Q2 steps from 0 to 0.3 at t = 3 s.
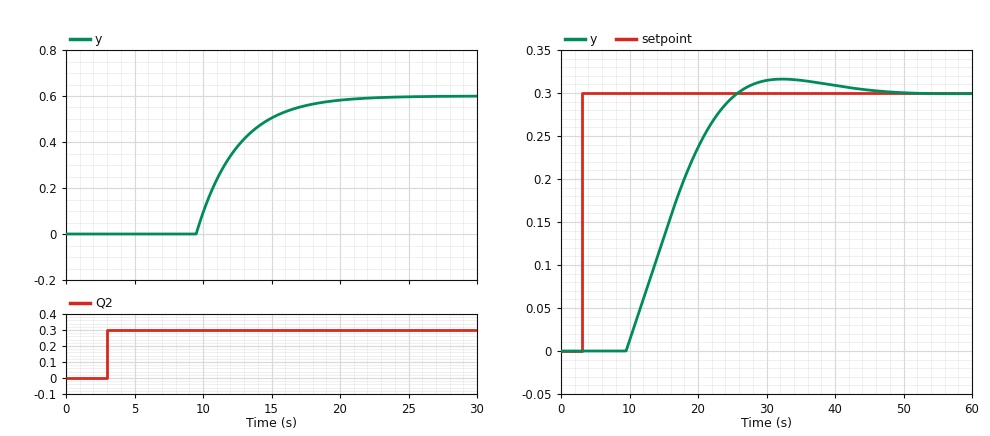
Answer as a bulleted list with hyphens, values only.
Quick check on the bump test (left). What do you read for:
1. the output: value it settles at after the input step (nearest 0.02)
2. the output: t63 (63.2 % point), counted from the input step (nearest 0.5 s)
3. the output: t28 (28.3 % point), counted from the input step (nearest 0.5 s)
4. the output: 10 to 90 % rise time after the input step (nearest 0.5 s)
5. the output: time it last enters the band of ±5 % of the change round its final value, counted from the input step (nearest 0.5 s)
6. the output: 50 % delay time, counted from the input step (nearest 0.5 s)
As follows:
- 0.60
- 9.5 s
- 7.5 s
- 6.5 s
- 15.5 s
- 8.5 s
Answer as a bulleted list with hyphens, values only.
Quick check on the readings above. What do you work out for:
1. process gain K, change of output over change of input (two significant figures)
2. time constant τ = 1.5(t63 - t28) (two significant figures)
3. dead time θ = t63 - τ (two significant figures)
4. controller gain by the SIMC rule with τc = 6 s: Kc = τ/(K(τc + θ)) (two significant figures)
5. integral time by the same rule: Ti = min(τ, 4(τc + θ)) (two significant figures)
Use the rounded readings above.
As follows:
- 2.0
- 3.0 s
- 6.5 s
- 0.12
- 3.0 s
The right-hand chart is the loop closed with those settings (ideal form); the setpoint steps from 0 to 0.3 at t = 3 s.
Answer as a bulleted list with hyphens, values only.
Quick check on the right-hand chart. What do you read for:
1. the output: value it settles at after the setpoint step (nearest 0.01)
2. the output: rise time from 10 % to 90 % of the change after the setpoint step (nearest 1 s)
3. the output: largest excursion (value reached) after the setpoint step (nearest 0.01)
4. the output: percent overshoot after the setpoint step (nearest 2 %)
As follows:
- 0.30
- 12 s
- 0.32
- 6 %
